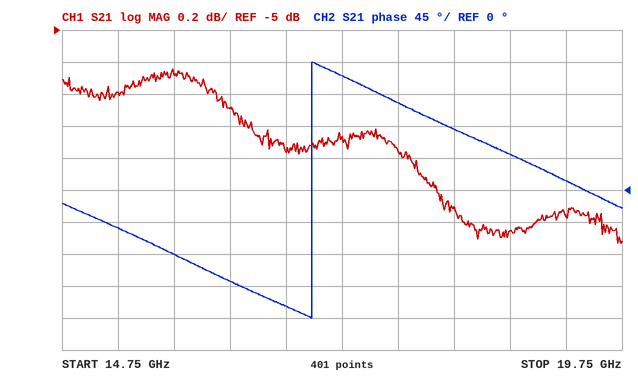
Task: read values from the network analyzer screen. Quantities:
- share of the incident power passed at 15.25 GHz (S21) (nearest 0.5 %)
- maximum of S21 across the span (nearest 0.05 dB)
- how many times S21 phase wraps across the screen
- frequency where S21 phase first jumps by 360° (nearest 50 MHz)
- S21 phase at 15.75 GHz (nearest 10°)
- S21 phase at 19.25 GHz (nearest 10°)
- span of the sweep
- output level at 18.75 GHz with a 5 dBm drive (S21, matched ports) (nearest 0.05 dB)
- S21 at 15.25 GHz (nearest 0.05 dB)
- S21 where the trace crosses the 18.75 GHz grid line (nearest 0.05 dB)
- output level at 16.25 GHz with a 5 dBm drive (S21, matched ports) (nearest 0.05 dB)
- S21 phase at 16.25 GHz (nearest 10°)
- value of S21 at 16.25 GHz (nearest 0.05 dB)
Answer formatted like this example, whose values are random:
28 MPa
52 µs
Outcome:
29.0 %
-5.25 dB
1
17.00 GHz
-90°
10°
5 GHz
-1.25 dBm
-5.40 dB
-6.25 dB
-0.50 dBm
-130°
-5.50 dB
